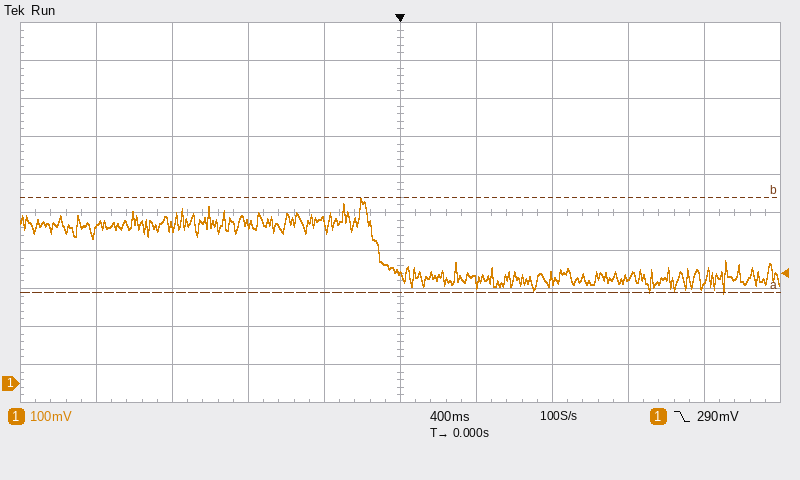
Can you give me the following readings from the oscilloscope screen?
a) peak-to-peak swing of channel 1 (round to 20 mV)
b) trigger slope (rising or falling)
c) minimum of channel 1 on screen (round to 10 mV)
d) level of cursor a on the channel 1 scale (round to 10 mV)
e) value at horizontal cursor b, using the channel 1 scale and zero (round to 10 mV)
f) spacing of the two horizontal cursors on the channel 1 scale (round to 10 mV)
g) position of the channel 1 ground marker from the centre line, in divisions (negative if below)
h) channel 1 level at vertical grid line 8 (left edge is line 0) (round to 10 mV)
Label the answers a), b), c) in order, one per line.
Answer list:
a) 240 mV
b) falling
c) 240 mV
d) 240 mV
e) 490 mV
f) 250 mV
g) -4.5 div
h) 280 mV
